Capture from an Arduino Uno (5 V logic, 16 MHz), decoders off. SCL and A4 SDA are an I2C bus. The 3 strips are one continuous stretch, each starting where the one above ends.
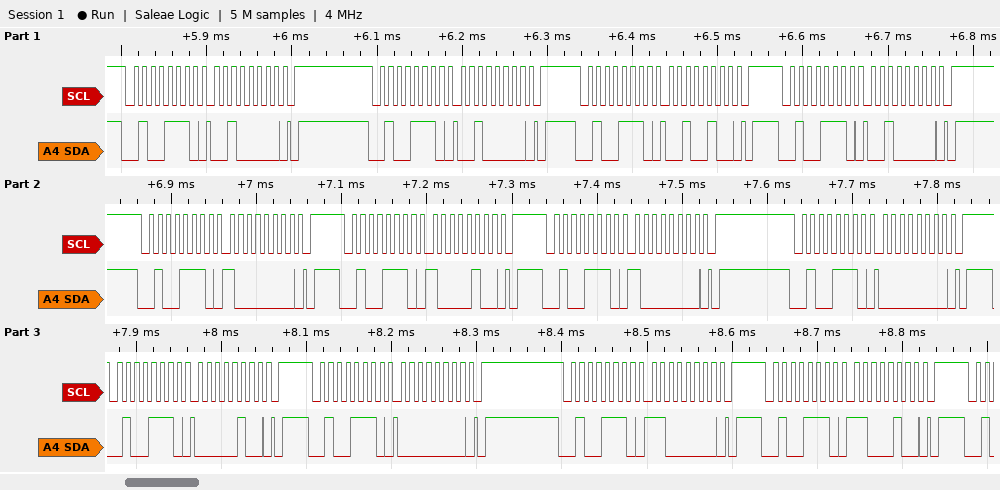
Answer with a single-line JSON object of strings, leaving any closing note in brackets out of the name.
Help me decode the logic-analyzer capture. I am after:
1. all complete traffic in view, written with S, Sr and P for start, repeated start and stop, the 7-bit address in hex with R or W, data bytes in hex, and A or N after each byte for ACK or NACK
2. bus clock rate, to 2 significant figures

{"all complete traffic in view, written with S, Sr and P for start, repeated start and stop, the 7-bit address in hex with R or W, data bytes in hex, and A or N after each byte for ACK or NACK": "S 27W A 20 A P S 27W A 20 A P S 27W A 24 A P S 27W A 20 A P S 27W A 80 A P S 27W A 84 A P S 27W A 80 A P S 27W A 00 A P S 27W A 04 A P S 27W A 00 A P S 27W A C0 A P S 27W A C4 A P", "bus clock rate, to 2 significant figures": "100 kHz"}
